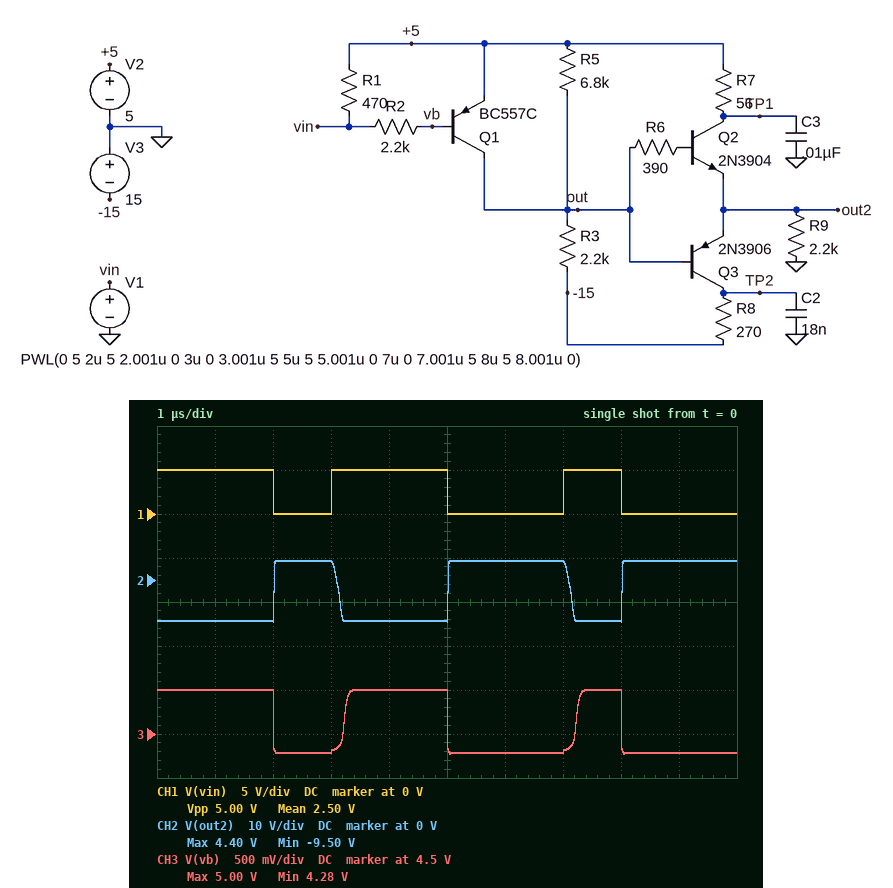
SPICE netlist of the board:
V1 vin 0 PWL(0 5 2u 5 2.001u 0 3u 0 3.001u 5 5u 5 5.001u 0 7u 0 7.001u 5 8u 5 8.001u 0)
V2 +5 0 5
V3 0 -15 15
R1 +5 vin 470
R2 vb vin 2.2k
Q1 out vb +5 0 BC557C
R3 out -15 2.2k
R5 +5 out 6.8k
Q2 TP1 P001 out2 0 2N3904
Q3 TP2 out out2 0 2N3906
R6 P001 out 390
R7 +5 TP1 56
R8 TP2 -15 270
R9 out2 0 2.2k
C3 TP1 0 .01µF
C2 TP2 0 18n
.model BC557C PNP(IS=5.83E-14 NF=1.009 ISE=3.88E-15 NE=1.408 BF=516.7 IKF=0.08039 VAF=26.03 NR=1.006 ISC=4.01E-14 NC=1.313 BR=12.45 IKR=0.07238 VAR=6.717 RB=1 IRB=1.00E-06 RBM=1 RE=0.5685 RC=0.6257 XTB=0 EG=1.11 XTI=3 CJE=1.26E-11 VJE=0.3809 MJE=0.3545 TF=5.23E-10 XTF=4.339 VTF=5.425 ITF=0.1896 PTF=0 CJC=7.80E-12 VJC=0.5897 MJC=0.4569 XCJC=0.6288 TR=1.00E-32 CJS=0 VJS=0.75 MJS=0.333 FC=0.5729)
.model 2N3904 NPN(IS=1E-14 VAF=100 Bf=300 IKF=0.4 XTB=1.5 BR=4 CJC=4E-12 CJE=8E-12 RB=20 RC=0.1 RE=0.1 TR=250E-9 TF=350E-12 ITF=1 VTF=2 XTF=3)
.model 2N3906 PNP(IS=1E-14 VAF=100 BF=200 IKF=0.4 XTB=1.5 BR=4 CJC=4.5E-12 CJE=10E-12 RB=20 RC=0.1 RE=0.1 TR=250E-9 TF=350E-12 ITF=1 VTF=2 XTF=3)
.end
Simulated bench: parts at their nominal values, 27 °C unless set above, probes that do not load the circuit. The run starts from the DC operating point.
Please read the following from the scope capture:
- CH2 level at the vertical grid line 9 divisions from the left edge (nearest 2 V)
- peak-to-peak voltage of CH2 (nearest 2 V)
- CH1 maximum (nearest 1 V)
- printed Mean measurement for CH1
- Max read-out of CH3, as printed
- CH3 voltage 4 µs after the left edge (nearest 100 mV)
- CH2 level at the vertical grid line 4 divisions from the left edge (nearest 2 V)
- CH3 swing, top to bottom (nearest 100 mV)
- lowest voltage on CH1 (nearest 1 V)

4 V
14 V
5 V
2.50 V
5.00 V
5.0 V
-10 V
700 mV
0 V
